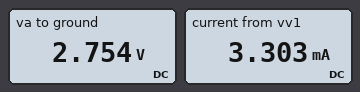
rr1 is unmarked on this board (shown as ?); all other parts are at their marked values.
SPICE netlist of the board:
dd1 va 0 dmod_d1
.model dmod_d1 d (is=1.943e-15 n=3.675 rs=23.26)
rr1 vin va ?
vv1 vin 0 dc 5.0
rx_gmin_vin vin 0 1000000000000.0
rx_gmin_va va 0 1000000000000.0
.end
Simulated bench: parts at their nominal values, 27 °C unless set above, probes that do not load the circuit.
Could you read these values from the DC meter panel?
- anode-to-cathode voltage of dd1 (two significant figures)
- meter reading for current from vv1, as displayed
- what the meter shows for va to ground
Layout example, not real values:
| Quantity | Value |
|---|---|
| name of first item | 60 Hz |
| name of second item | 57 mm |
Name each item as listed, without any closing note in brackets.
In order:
| Quantity | Value |
|---|---|
| anode-to-cathode voltage of dd1 | 2.8 V |
| meter reading for current from vv1, as displayed | 3.303 mA |
| what the meter shows for va to ground | 2.754 V |
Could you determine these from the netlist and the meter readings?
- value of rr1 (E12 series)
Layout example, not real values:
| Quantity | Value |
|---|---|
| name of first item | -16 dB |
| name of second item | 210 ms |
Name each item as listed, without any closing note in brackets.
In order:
| Quantity | Value |
|---|---|
| value of rr1 | 680 Ω |
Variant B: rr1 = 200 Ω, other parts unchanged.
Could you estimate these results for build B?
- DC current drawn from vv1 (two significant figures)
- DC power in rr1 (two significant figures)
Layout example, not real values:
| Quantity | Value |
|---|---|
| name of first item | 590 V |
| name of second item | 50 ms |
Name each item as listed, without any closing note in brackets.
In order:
| Quantity | Value |
|---|---|
| DC current drawn from vv1 | 9.9 mA |
| DC power in rr1 | 20 mW |
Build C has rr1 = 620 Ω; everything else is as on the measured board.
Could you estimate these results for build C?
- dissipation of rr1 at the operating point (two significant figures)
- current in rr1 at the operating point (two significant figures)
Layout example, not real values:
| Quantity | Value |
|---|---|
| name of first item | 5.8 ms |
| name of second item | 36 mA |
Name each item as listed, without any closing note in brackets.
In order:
| Quantity | Value |
|---|---|
| dissipation of rr1 at the operating point | 8.0 mW |
| current in rr1 at the operating point | 3.6 mA |
